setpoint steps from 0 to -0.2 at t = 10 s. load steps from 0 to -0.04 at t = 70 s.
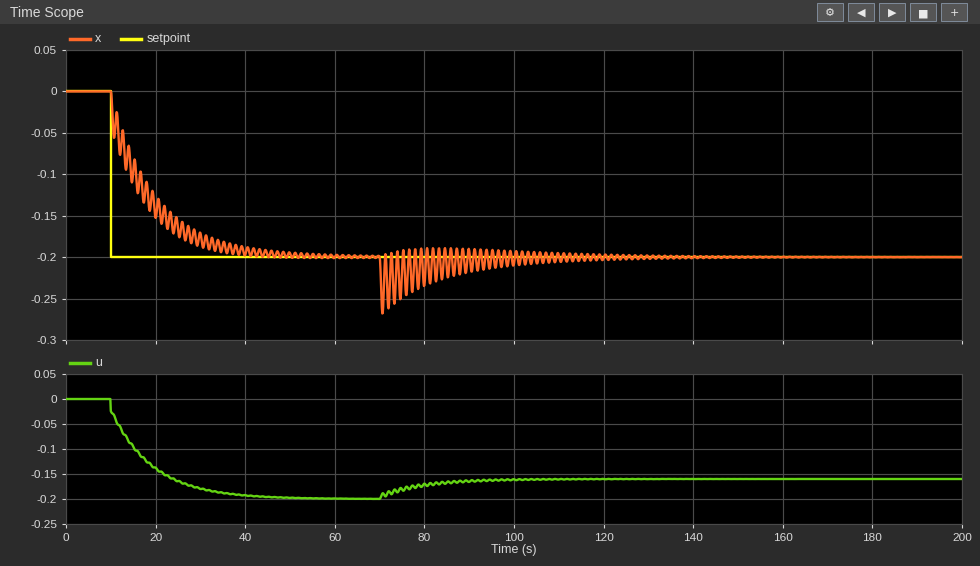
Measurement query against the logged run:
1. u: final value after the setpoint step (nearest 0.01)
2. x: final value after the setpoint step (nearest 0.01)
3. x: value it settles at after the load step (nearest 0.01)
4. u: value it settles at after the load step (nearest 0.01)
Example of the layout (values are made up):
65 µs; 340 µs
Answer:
-0.20; -0.20; -0.20; -0.16
